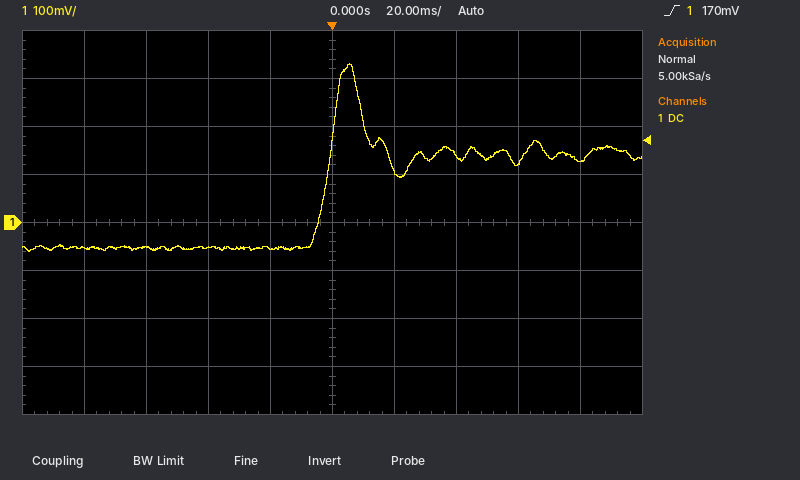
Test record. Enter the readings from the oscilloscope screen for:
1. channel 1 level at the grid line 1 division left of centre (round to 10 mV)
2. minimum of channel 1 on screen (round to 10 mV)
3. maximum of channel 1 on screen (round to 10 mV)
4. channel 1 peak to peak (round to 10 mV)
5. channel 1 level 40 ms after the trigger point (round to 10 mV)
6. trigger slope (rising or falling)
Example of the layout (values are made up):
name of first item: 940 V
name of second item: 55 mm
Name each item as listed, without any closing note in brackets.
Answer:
channel 1 level at the grid line 1 division left of centre: -50 mV
minimum of channel 1 on screen: -60 mV
maximum of channel 1 on screen: 330 mV
channel 1 peak to peak: 390 mV
channel 1 level 40 ms after the trigger point: 140 mV
trigger slope: rising
